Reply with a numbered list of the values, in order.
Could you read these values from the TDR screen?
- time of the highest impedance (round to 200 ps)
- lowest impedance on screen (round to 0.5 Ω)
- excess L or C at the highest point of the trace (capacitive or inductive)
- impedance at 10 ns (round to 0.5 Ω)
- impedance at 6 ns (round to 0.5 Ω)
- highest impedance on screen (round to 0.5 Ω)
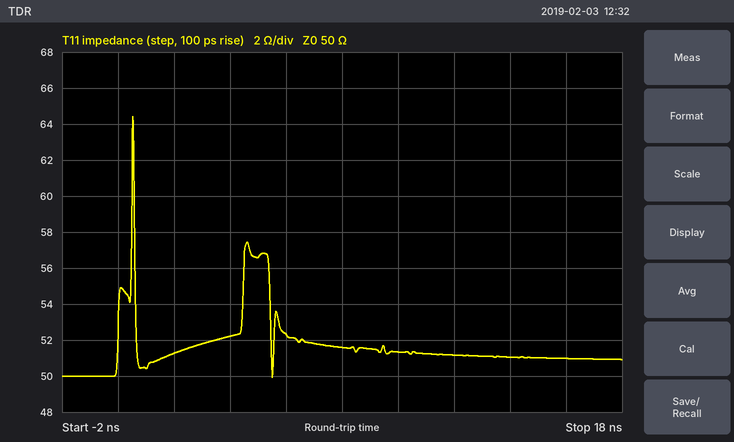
1. 600 ps
2. 50.0 Ω
3. inductive
4. 51.5 Ω
5. 52.5 Ω
6. 64.5 Ω
